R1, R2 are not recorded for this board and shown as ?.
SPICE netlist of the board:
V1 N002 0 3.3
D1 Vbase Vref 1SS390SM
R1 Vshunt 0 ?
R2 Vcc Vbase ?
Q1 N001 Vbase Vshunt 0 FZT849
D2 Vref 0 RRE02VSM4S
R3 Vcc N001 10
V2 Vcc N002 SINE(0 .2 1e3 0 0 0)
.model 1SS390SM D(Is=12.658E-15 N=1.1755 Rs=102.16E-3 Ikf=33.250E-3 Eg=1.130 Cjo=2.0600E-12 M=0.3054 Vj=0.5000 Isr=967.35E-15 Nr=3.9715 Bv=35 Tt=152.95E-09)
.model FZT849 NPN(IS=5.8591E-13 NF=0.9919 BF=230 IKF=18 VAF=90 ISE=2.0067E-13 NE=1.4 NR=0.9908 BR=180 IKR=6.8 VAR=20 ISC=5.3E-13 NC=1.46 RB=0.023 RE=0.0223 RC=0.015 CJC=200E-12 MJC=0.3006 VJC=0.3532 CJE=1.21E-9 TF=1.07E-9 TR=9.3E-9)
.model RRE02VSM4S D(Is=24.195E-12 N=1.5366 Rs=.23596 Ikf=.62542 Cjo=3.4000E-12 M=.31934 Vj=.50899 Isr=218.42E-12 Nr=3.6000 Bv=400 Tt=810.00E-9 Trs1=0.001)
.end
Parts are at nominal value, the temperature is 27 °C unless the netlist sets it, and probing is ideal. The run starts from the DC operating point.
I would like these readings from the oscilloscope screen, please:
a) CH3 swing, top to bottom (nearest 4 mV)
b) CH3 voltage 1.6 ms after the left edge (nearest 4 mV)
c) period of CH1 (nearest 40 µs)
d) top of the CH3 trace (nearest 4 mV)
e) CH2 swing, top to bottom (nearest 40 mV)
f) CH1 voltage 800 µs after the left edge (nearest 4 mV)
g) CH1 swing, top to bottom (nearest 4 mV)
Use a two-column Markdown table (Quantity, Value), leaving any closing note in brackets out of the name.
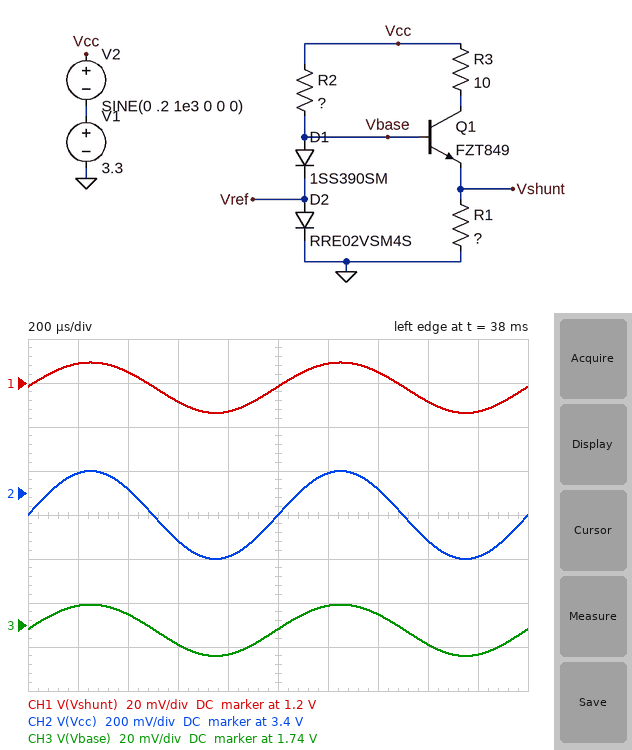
| Quantity | Value |
|---|---|
| CH3 swing, top to bottom | 24 mV |
| CH3 voltage 1.6 ms after the left edge | 1.732 V |
| period of CH1 | 1.00 ms |
| top of the CH3 trace | 1.748 V |
| CH2 swing, top to bottom | 400 mV |
| CH1 voltage 800 µs after the left edge | 1.188 V |
| CH1 swing, top to bottom | 24 mV |
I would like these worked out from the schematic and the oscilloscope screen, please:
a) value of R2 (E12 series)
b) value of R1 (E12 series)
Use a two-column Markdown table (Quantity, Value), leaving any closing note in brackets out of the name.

| Quantity | Value |
|---|---|
| value of R2 | 56 Ω |
| value of R1 | 1.5 kΩ |
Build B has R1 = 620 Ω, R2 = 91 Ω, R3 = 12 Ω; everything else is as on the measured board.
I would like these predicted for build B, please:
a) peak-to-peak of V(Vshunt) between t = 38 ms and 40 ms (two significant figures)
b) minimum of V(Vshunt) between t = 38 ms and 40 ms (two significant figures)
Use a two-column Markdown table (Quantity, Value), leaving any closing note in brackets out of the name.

| Quantity | Value |
|---|---|
| peak-to-peak of V(Vshunt) between t = 38 ms and 40 ms | 21 mV |
| minimum of V(Vshunt) between t = 38 ms and 40 ms | 1.1 V |
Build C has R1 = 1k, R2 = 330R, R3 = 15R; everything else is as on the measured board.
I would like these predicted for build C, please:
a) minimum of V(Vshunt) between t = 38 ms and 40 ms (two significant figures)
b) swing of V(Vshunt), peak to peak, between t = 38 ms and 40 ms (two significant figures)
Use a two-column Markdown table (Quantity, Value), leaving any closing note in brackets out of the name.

| Quantity | Value |
|---|---|
| minimum of V(Vshunt) between t = 38 ms and 40 ms | 1.0 V |
| swing of V(Vshunt), peak to peak, between t = 38 ms and 40 ms | 18 mV |
